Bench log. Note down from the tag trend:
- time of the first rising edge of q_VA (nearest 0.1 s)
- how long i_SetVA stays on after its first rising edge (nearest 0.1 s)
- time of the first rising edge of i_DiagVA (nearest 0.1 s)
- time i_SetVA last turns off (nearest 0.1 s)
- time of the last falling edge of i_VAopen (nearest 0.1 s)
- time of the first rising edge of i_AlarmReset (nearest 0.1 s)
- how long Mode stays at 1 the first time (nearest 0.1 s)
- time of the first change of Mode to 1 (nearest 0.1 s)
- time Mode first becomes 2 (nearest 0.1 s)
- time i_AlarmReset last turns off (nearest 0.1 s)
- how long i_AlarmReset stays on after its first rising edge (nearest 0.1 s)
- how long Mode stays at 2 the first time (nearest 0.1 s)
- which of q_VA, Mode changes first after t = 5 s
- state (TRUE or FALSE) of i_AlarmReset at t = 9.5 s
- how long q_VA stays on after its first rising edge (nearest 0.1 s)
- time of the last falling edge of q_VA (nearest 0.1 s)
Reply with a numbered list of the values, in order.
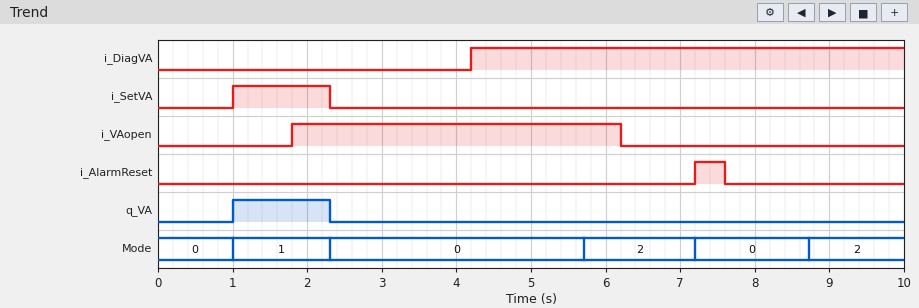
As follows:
1. 1.0 s
2. 1.3 s
3. 4.2 s
4. 2.3 s
5. 6.2 s
6. 7.2 s
7. 1.3 s
8. 1.0 s
9. 5.7 s
10. 7.6 s
11. 0.4 s
12. 1.5 s
13. Mode
14. FALSE
15. 1.3 s
16. 2.3 s
